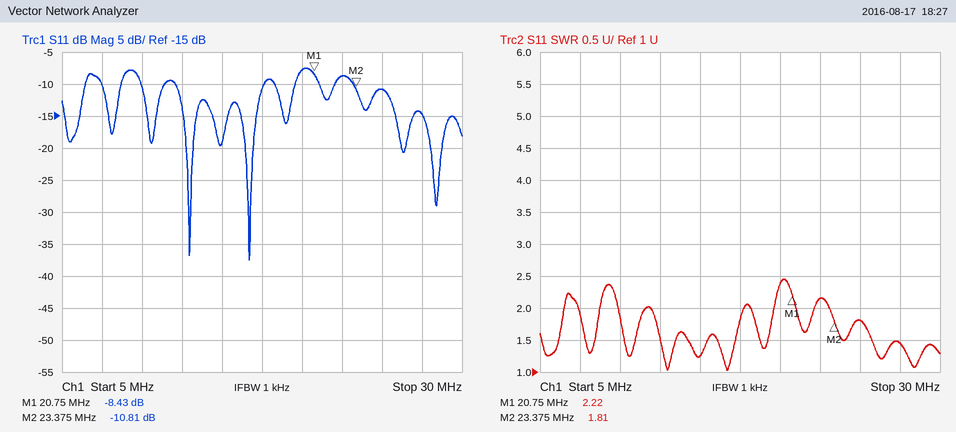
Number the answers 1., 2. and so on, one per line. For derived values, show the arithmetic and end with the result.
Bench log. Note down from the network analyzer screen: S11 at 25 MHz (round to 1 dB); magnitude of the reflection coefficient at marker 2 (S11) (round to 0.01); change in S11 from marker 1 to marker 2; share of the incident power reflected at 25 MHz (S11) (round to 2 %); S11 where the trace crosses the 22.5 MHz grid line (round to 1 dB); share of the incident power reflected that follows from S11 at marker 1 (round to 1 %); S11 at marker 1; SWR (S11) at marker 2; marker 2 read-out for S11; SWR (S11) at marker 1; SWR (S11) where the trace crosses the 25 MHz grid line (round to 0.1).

1. -11 dB
2. 10^(-10.81/20) ≈ 0.29
3. -10.81 − (-8.43) = -2.38 dB
4. 10^(-11/10) ≈ 8 %
5. -9 dB
6. 10^(-8.43/10) ≈ 14 %
7. -8.43 dB
8. 1.81
9. -10.81 dB
10. 2.22
11. 1.8
